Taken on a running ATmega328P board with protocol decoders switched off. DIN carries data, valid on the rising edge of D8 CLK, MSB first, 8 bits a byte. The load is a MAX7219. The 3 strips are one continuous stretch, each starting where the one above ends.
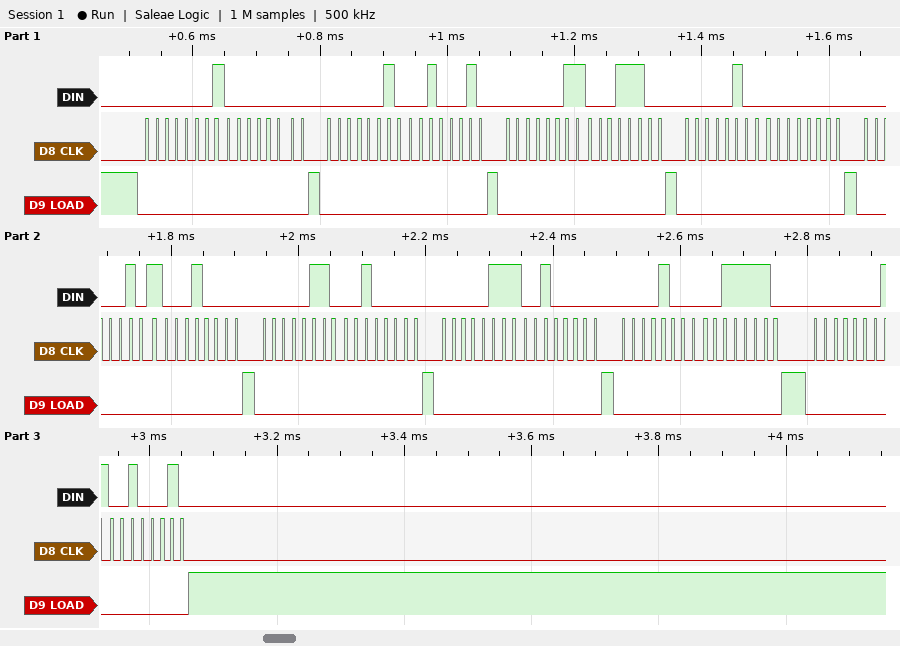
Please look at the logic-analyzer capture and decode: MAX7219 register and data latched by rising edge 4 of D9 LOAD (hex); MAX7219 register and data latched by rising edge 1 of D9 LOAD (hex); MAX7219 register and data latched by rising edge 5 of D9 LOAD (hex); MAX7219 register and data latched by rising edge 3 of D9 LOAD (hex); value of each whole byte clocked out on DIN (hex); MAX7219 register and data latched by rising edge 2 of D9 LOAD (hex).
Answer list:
register 0x4, data 0x00
register 0x1, data 0x00
register 0x5, data 0x10
register 0x3, data 0x1C
01 00 02 22 03 1C 04 00 05 10 06 20 07 20 08 3E 01 22
register 0x2, data 0x22
